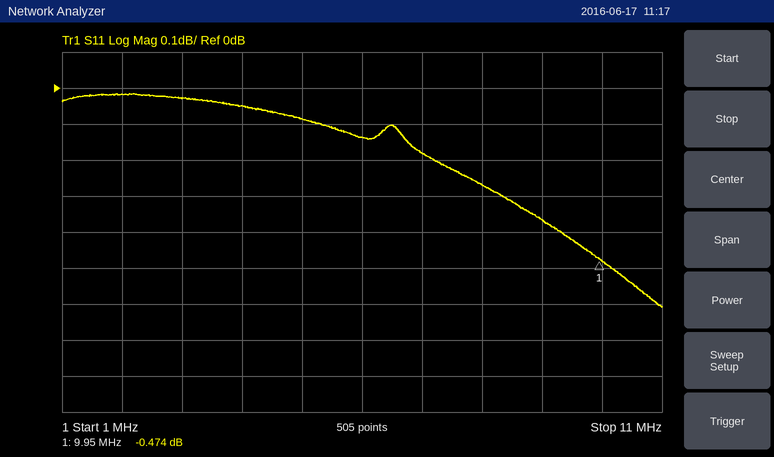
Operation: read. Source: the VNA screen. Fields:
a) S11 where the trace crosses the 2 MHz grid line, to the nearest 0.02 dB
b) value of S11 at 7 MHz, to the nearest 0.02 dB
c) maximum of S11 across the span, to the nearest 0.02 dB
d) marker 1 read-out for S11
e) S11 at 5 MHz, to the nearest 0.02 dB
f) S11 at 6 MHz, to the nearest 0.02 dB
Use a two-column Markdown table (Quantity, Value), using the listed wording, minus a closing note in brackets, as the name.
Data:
| Quantity | Value |
|---|---|
| S11 where the trace crosses the 2 MHz grid line, to the nearest 0.02 dB | -0.02 dB |
| value of S11 at 7 MHz, to the nearest 0.02 dB | -0.18 dB |
| maximum of S11 across the span, to the nearest 0.02 dB | -0.02 dB |
| marker 1 read-out for S11 | -0.474 dB |
| S11 at 5 MHz, to the nearest 0.02 dB | -0.08 dB |
| S11 at 6 MHz, to the nearest 0.02 dB | -0.14 dB |
